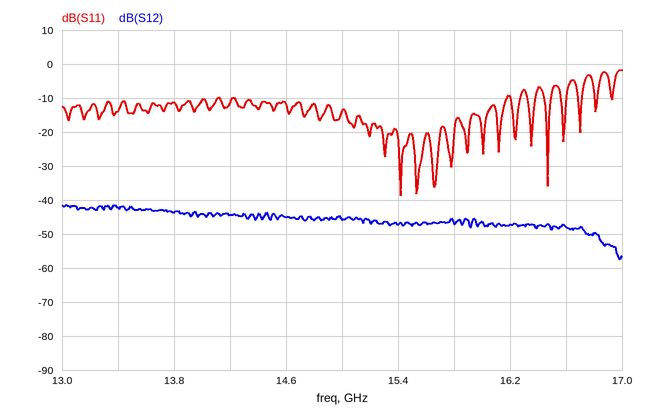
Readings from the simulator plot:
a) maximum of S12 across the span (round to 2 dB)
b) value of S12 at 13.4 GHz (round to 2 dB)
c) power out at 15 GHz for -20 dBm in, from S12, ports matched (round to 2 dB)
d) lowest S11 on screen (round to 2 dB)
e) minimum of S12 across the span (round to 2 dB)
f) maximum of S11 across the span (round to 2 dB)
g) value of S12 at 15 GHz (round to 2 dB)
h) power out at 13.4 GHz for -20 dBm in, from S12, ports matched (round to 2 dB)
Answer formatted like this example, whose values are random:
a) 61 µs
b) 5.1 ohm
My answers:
a) -42 dB
b) -42 dB
c) -66 dBm
d) -38 dB
e) -58 dB
f) -2 dB
g) -46 dB
h) -62 dBm
